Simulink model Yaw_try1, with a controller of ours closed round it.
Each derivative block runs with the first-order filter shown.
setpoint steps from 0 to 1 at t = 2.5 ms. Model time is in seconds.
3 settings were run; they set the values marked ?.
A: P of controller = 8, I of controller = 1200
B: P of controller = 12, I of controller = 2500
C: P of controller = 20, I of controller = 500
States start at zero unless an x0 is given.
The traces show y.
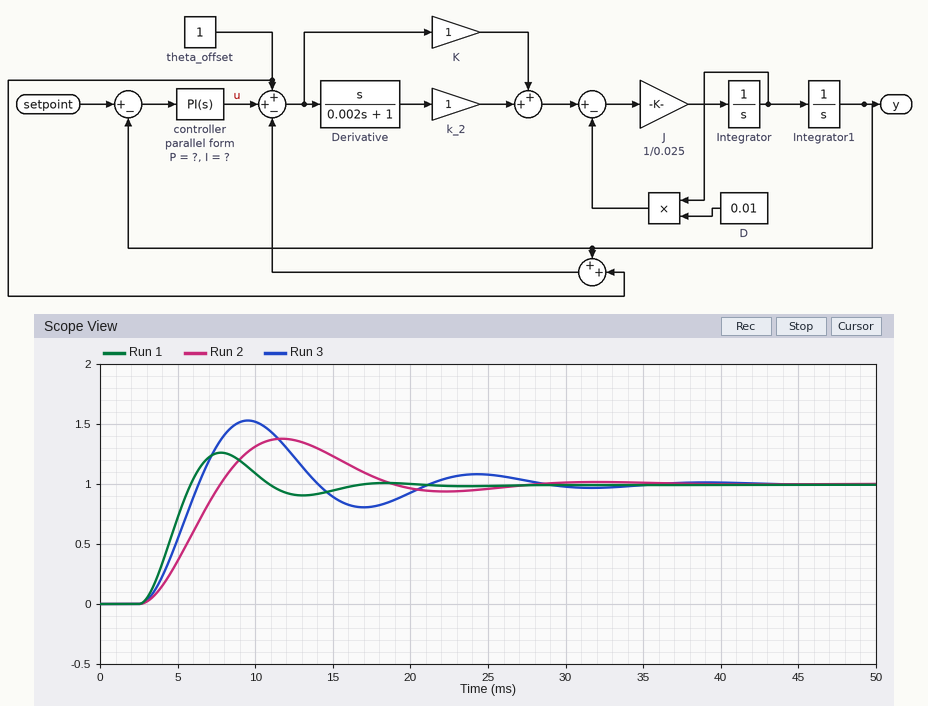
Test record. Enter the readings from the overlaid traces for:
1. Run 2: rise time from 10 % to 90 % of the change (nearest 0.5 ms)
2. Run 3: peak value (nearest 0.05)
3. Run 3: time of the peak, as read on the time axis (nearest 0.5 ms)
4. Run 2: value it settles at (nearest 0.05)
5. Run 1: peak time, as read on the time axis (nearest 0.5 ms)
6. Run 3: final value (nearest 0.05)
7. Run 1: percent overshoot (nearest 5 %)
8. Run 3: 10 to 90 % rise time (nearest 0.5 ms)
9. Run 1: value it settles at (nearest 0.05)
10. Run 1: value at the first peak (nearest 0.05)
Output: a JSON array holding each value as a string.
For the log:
["3.5 ms", "1.55", "9.5 ms", "1.00", "8.0 ms", "1.00", "25 %", "2.5 ms", "1.00", "1.25"]
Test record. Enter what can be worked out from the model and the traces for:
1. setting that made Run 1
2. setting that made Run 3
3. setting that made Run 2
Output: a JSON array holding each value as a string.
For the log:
["C", "B", "A"]
